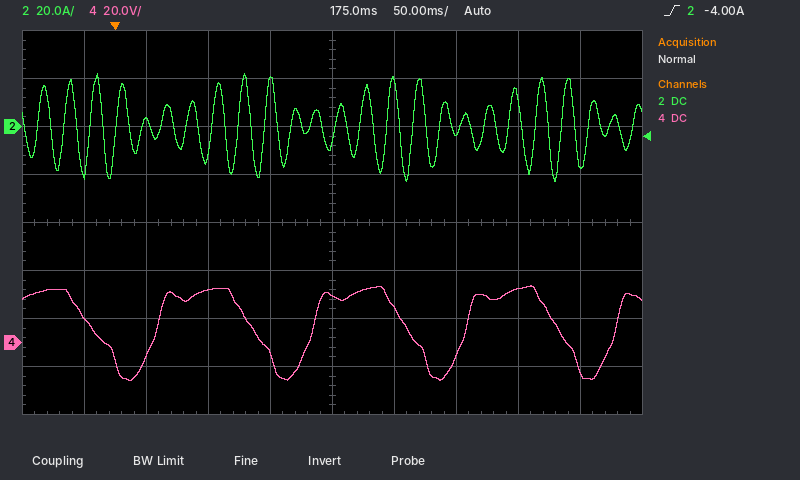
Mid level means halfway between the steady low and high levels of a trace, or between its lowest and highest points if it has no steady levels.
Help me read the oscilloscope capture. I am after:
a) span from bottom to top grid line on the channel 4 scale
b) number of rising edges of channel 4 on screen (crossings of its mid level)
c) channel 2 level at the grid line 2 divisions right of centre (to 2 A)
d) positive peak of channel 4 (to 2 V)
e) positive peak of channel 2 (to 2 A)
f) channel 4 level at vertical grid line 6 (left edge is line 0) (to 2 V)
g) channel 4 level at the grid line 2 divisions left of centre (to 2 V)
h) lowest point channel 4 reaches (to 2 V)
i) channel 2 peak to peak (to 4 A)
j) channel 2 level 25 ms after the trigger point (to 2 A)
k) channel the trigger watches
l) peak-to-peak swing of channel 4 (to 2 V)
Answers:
160 V
4
-2 A
24 V
22 A
14 V
22 V
-16 V
44 A
2 A
channel 2
40 V
